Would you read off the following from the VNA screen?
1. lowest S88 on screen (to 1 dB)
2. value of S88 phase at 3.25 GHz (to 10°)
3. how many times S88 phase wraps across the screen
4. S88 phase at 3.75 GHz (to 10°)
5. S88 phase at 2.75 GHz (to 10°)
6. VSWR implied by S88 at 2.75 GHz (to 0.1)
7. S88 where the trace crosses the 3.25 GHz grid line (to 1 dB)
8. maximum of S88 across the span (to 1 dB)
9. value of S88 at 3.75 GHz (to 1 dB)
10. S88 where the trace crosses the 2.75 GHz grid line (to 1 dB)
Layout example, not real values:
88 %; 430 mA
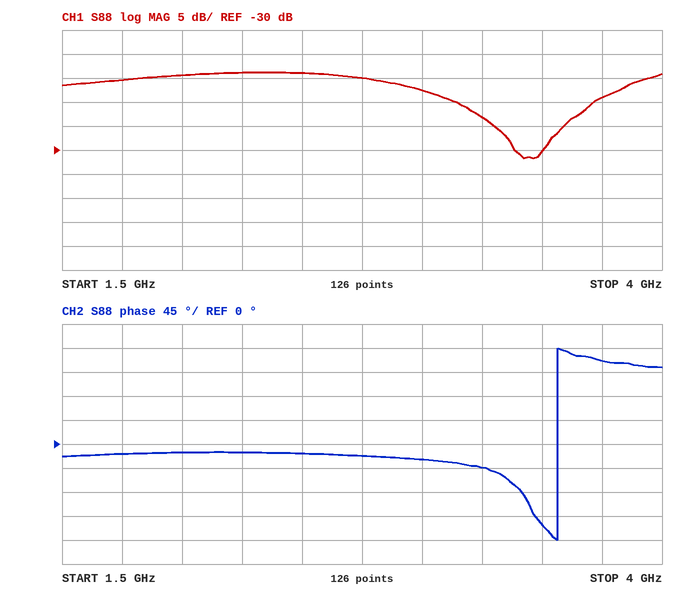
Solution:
-32 dB; -40°; 1; 160°; -20°; 1.4; -23 dB; -14 dB; -19 dB; -15 dB
